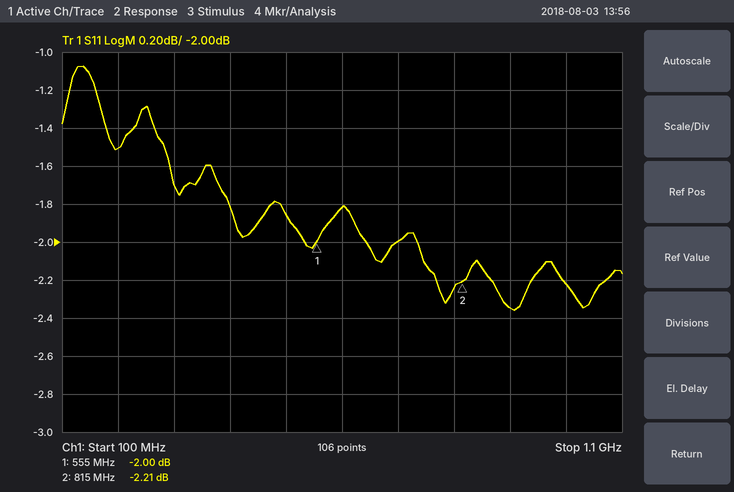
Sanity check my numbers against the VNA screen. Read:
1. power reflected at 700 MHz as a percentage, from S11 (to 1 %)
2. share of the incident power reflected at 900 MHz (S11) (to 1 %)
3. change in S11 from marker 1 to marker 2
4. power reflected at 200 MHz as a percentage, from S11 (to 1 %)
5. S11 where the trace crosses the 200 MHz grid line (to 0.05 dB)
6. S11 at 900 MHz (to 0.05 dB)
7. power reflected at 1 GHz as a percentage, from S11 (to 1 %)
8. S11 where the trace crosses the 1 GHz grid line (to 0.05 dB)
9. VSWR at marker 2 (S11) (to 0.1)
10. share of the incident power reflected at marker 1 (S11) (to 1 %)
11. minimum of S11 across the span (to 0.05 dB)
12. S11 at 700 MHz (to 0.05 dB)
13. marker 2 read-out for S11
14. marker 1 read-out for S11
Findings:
63 %
58 %
-0.21 dB
71 %
-1.50 dB
-2.35 dB
60 %
-2.20 dB
7.9
63 %
-2.35 dB
-2.00 dB
-2.21 dB
-2.00 dB
